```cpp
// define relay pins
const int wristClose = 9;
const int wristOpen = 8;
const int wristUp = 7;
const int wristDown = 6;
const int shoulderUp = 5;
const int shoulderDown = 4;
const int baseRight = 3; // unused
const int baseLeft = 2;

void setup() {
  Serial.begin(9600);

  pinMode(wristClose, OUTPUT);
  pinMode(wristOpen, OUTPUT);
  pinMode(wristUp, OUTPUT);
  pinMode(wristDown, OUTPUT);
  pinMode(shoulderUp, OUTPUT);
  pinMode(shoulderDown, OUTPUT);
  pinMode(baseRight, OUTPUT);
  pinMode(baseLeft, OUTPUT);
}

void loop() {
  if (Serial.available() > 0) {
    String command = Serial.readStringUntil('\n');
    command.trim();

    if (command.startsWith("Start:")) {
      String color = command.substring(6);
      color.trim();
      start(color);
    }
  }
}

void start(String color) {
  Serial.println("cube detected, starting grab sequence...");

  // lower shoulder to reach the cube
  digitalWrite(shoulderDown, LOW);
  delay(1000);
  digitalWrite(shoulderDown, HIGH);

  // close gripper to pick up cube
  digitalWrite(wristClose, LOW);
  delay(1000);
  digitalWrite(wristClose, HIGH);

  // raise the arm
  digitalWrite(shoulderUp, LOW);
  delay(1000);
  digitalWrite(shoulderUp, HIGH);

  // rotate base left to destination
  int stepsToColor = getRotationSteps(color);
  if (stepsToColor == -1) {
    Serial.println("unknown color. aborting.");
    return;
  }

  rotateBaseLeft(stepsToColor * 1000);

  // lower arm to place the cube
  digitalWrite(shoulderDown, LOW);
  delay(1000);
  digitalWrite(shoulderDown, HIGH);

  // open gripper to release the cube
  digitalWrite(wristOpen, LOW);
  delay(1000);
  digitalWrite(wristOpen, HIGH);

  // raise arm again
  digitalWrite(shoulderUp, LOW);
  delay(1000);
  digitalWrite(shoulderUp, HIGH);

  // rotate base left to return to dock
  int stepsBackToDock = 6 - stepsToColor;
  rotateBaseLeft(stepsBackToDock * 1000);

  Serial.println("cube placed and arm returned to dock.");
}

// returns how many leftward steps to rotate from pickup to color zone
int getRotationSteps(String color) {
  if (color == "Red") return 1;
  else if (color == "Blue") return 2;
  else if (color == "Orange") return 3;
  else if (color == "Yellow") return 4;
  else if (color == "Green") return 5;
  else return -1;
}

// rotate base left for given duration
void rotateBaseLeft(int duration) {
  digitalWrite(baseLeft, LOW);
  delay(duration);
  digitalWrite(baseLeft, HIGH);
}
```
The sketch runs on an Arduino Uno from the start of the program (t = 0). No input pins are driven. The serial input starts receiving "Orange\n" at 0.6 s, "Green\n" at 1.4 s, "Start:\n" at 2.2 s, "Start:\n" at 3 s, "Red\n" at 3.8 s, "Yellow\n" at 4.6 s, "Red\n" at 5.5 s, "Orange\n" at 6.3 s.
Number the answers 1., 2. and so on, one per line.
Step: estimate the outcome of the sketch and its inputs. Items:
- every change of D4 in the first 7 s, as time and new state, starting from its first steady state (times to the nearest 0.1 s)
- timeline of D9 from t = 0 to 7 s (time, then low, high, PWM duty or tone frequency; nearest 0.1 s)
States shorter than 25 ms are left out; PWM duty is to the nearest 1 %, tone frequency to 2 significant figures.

1. 0 s low; 3.2 s high; 5.2 s low; 6.2 s high
2. 0 s low; 4.2 s high; 6.2 s low
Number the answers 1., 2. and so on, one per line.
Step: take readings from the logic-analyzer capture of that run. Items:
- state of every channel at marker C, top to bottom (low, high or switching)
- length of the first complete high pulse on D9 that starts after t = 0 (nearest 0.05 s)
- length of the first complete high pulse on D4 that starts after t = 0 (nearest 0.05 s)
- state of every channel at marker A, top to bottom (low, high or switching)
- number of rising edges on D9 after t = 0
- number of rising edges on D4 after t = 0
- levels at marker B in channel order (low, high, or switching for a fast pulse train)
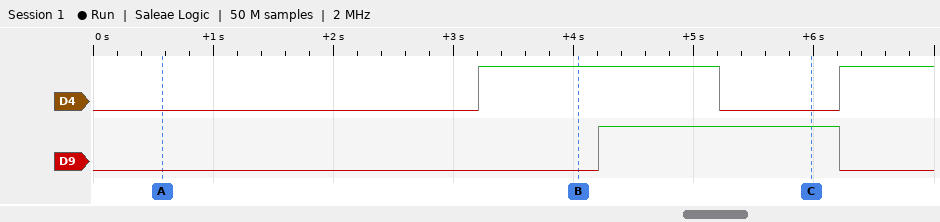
1. D4 low, D9 high
2. 2.00 s
3. 2.00 s
4. D4 low, D9 low
5. 1
6. 2
7. D4 high, D9 low
